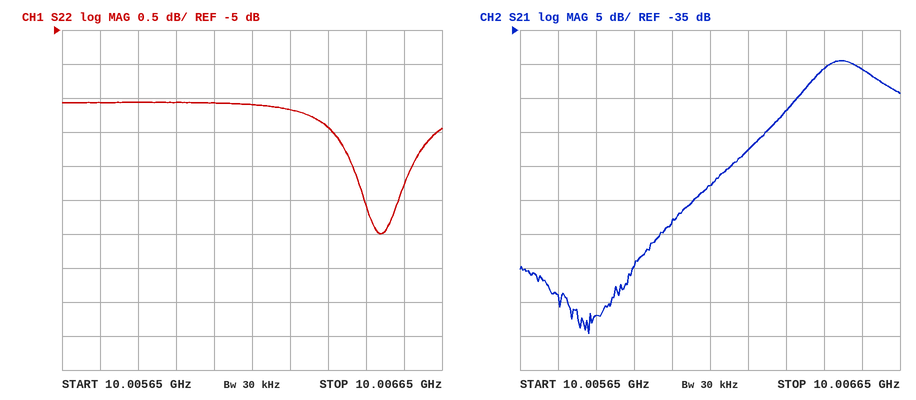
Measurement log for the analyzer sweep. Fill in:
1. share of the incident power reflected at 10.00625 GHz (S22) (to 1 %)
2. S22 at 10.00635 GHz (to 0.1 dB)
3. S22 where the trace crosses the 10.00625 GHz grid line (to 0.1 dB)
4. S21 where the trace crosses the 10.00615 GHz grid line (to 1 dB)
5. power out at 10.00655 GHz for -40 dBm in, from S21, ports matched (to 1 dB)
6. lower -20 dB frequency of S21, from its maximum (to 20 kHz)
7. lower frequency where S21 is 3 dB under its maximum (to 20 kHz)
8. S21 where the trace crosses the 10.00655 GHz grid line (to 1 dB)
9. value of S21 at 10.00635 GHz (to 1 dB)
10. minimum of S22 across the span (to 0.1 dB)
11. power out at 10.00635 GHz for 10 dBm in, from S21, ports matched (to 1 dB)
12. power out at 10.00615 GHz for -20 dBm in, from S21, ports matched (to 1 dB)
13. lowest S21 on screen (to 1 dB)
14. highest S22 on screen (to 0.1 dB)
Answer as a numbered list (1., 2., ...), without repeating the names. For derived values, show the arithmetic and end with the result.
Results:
1. 10^(-6.2/10) ≈ 24 %
2. -6.4 dB
3. -6.2 dB
4. -58 dB
5. -40 dBm + (-41 dB) = -81 dBm
6. 10.00612 GHz
7. 10.00642 GHz
8. -41 dB
9. -47 dB
10. -8.0 dB
11. 10 dBm + (-47 dB) = -37 dBm
12. -20 dBm + (-58 dB) = -78 dBm
13. -80 dB
14. -6.1 dB
